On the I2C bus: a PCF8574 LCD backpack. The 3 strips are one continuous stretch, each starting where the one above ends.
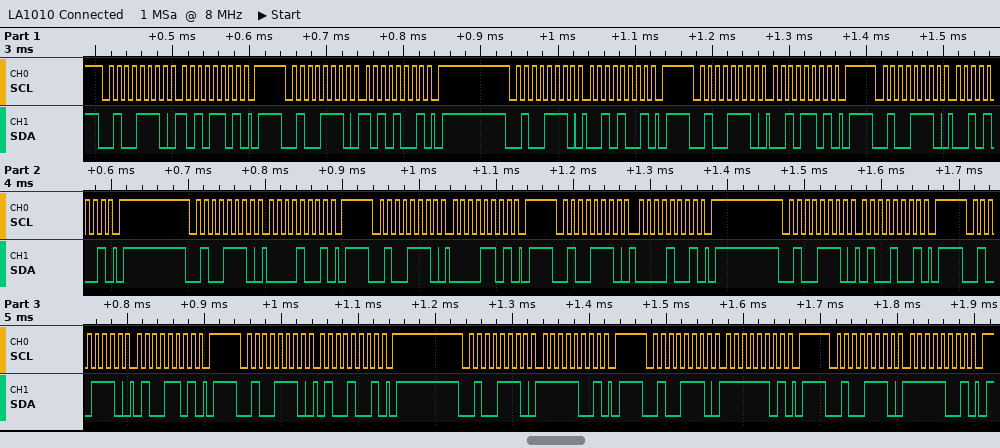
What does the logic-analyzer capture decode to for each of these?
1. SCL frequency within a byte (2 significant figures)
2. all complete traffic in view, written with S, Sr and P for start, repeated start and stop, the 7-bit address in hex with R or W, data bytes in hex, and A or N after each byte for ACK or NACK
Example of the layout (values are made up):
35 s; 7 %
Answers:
100 kHz; S 27W A AD A P S 27W A A9 A P S 27W A 29 A P S 27W A 2D A P S 27W A 29 A P S 27W A 09 A P S 27W A 0D A P S 27W A 09 A P S 27W A 49 A P S 27W A 4D A P S 27W A 49 A P S 27W A F9 A P S 27W A FD A P S 27W A F9 A P
